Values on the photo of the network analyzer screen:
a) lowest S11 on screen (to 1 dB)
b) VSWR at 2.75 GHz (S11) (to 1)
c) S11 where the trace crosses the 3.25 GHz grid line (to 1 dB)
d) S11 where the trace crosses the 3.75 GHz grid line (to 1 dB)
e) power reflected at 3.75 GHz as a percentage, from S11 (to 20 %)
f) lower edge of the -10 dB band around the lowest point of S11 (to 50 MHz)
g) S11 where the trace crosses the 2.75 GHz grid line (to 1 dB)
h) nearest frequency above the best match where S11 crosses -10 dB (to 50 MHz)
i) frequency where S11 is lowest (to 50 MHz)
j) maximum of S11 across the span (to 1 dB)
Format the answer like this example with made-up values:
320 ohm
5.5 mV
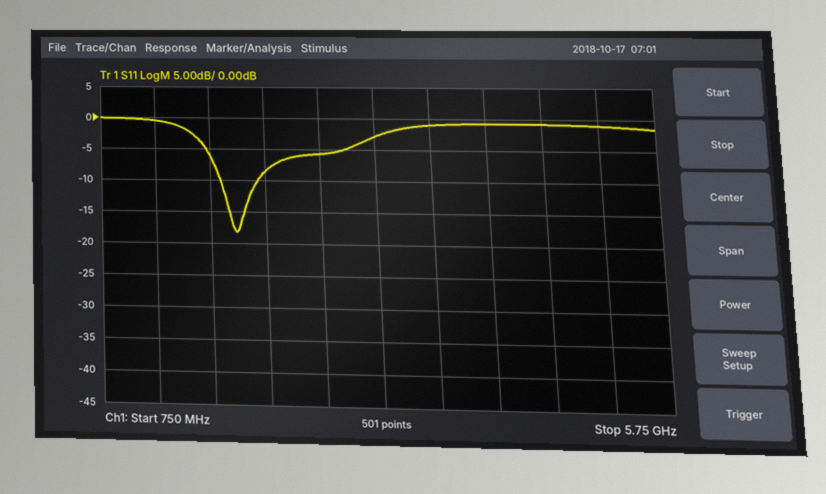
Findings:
-18 dB
3
-3 dB
-1 dB
80 %
1.85 GHz
-6 dB
2.20 GHz
2.00 GHz
0 dB
